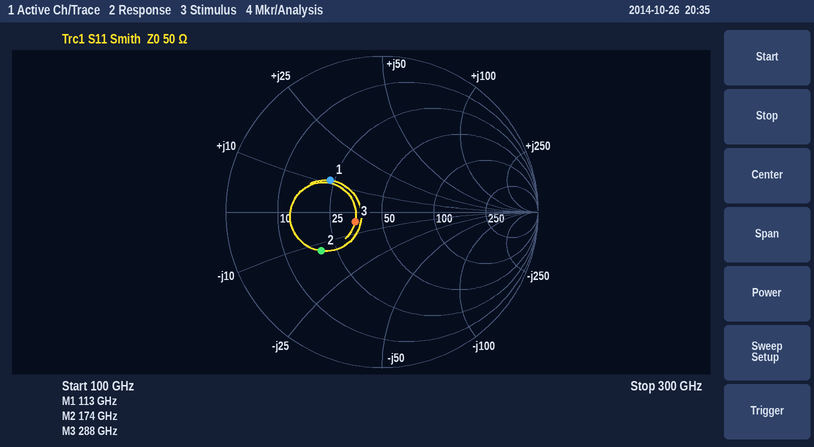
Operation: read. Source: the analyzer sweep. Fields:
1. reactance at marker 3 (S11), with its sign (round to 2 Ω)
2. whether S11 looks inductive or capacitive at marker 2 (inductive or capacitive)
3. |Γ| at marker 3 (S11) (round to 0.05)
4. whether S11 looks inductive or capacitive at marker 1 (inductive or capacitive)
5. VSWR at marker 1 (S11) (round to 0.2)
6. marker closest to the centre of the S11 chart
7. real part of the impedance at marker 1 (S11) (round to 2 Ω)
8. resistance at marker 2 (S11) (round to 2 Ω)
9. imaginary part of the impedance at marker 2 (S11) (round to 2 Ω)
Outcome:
-4 Ω
capacitive
0.20
inductive
2.2
marker 3
24 Ω
20 Ω
-12 Ω
